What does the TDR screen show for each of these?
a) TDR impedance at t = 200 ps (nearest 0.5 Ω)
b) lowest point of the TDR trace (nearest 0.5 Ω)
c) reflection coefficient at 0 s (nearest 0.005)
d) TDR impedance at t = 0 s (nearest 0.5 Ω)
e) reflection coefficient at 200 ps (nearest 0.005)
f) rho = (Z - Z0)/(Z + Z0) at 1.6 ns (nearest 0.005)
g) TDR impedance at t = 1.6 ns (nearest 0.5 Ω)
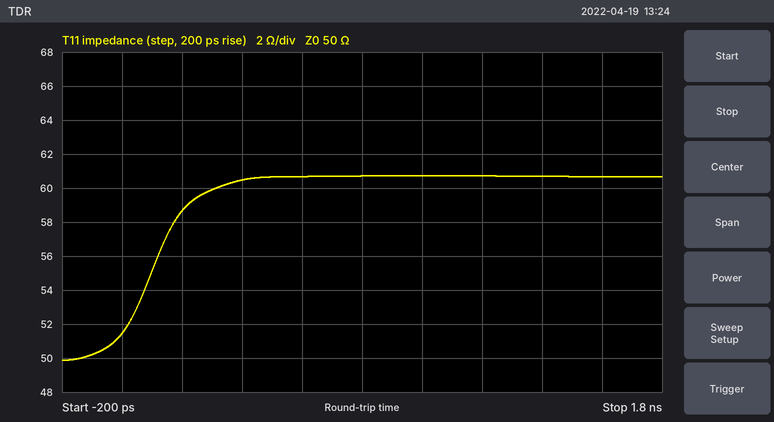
58.5 Ω
50.0 Ω
+0.015
51.5 Ω
+0.080
+0.095
60.5 Ω
